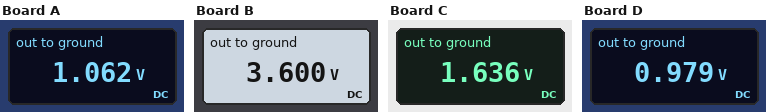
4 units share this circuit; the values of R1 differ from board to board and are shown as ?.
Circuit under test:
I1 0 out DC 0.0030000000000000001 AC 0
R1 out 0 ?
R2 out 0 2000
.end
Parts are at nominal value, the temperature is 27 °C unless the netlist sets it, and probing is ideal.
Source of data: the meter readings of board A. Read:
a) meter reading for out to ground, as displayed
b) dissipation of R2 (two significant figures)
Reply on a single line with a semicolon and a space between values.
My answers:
1.062 V; 560 µW
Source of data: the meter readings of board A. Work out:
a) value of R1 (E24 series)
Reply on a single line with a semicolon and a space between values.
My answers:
430 Ω
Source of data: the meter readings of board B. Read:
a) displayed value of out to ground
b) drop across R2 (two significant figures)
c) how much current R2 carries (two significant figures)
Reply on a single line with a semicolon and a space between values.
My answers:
3.600 V; 3.6 V; 1.8 mA
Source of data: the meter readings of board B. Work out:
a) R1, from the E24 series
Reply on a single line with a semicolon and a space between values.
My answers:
3 kΩ
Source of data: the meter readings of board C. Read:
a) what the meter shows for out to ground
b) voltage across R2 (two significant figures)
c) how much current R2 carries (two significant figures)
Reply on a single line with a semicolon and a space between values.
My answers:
1.636 V; 1.6 V; 820 µA
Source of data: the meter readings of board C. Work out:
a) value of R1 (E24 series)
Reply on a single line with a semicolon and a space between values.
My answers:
750 Ω
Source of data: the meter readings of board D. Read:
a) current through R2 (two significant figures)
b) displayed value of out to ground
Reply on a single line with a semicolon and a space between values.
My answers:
490 µA; 0.979 V
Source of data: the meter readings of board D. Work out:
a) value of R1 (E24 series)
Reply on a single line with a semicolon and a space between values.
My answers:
390 Ω
